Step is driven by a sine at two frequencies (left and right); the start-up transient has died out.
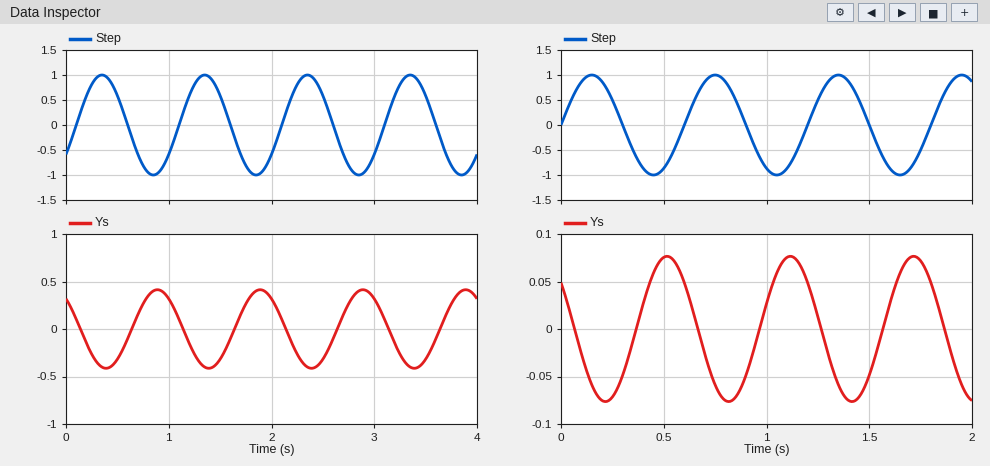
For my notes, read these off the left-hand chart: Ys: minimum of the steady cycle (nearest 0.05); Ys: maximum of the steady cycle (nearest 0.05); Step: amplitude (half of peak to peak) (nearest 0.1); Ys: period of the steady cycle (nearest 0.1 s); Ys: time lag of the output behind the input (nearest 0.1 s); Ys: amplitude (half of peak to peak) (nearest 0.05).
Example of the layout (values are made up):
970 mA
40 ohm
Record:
-0.40
0.40
1.0
1.0 s
0.5 s
0.40
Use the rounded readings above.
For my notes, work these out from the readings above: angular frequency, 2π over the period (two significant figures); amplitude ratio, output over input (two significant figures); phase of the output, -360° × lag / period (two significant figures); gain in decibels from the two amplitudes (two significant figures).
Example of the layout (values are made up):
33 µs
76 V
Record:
6.3 rad/s
0.40
-180°
-8.0 dB
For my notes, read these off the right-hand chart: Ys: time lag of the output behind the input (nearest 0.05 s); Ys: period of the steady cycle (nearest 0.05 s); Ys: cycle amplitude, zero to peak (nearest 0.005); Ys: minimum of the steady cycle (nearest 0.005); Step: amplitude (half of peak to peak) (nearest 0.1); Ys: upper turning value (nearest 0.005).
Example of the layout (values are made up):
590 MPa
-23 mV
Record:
0.35 s
0.60 s
0.075
-0.075
1.0
0.075
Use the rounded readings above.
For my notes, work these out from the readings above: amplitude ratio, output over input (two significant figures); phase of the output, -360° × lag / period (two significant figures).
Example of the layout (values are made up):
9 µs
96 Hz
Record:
0.075
-210°
